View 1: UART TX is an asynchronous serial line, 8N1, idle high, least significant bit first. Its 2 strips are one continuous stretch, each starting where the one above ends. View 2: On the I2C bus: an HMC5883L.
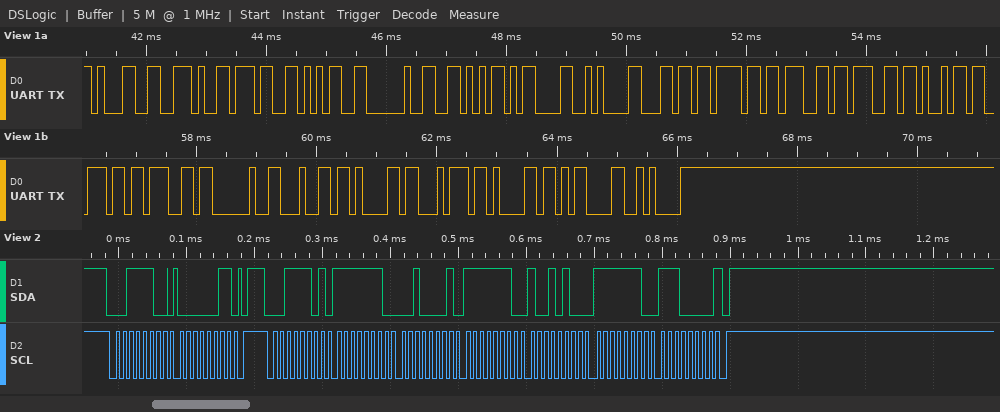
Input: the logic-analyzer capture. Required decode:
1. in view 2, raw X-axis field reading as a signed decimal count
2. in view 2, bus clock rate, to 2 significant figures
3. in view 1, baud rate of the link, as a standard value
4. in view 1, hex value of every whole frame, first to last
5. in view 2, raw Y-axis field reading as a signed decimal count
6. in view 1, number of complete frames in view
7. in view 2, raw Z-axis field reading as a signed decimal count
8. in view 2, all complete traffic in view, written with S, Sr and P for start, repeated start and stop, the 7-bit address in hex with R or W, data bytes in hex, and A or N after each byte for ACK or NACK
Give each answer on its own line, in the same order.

-479
100 kHz
9600 baud
0x31 0x2E 0x37 0x35 0x20 0x56 0x0D 0x0A 0x6C 0x6F 0x67 0x67 0x69 0x6E 0x67 0x20 0x64 0x61 0x74 0x61 0x0D 0x0A
-288
22
-364
S 1EW A 03 A P S 1ER A FE A 21 A FE A 94 A FE A E0 N P
